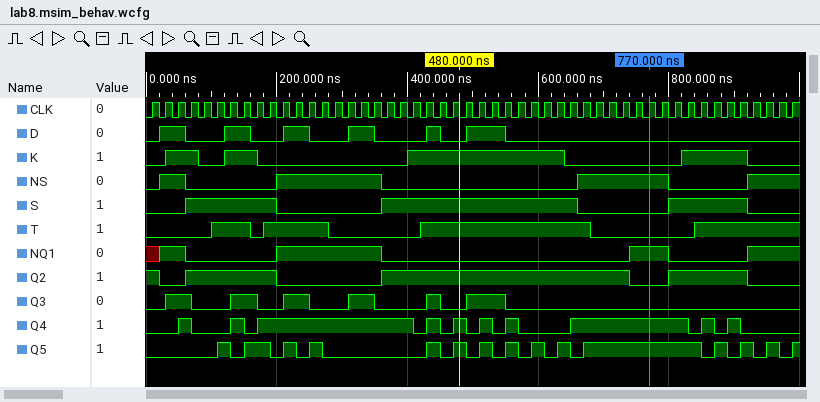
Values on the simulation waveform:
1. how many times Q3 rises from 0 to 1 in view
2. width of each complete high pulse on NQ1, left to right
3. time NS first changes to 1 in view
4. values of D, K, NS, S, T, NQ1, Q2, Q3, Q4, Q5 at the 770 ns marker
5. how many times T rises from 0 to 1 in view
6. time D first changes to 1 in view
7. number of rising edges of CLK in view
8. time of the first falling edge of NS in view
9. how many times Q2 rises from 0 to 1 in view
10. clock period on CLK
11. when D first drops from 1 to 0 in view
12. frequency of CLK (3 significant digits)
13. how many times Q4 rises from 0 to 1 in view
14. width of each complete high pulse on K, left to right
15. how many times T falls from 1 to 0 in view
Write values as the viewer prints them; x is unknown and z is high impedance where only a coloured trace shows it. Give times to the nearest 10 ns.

6
160 ns, 60 ns
20 ns
D=0, K=0, NS=1, S=0, T=0, NQ1=1, Q2=0, Q3=0, Q4=1, Q5=1
4
20 ns
50
60 ns
3
20 ns
60 ns
50.0 MHz
10
50 ns, 50 ns, 240 ns, 100 ns
3
